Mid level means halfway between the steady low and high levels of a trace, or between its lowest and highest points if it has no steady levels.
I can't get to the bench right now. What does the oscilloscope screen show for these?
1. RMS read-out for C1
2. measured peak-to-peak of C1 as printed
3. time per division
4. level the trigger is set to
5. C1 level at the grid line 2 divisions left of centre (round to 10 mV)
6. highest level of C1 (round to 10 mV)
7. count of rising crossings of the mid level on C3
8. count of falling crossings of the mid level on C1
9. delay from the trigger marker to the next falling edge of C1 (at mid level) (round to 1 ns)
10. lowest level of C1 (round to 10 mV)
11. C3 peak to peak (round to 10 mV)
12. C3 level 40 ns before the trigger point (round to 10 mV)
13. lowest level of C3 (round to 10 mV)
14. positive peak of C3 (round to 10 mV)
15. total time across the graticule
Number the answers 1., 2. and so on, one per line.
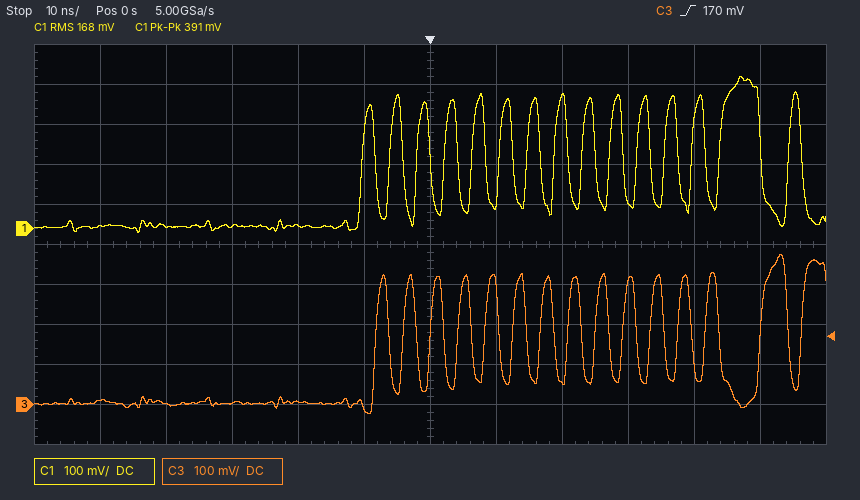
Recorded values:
1. 168 mV
2. 391 mV
3. 10 ns
4. 170 mV
5. 10 mV
6. 380 mV
7. 15
8. 15
9. 4 ns
10. -10 mV
11. 400 mV
12. 0 mV
13. -20 mV
14. 380 mV
15. 120 ns
